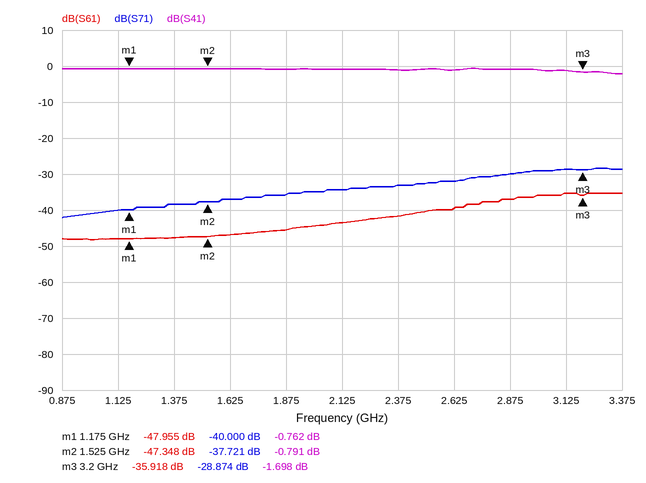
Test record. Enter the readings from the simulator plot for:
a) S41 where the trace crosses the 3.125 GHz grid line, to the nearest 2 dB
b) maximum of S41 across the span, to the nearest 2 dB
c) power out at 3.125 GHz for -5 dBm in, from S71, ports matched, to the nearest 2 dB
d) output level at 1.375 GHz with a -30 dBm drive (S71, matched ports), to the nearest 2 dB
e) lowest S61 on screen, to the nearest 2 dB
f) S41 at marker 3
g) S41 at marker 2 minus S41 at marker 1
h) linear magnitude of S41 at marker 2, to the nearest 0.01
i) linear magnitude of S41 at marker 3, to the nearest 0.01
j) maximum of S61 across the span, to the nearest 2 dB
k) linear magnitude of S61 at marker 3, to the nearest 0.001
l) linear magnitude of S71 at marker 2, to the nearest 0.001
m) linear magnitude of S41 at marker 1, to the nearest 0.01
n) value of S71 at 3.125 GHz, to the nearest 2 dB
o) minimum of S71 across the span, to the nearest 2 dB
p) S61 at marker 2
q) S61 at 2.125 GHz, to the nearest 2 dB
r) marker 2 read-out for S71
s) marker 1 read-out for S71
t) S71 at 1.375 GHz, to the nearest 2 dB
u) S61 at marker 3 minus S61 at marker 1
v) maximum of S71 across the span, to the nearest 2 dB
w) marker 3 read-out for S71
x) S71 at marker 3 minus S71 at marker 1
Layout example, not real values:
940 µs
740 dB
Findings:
-2 dB
0 dB
-34 dBm
-68 dBm
-48 dB
-1.698 dB
-0.029 dB
0.91
0.82
-36 dB
0.016
0.013
0.92
-28 dB
-42 dB
-47.348 dB
-44 dB
-37.721 dB
-40.000 dB
-38 dB
12.037 dB
-28 dB
-28.874 dB
11.126 dB
